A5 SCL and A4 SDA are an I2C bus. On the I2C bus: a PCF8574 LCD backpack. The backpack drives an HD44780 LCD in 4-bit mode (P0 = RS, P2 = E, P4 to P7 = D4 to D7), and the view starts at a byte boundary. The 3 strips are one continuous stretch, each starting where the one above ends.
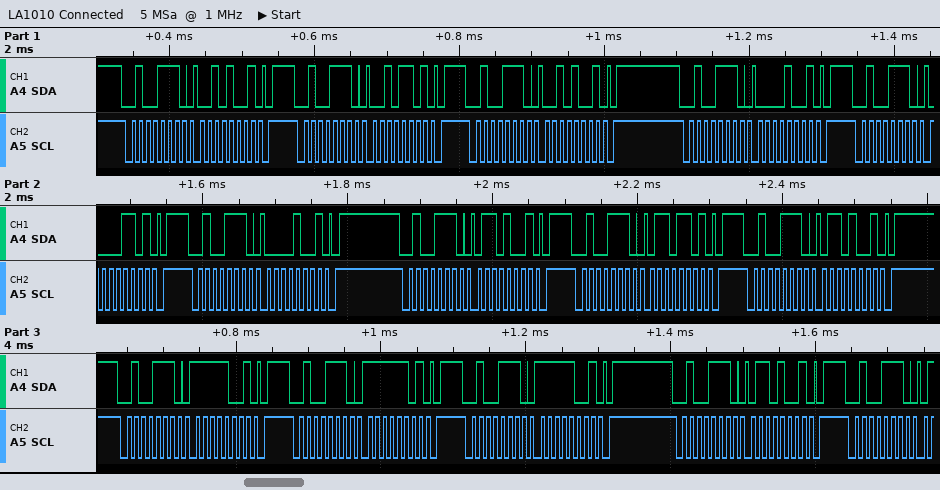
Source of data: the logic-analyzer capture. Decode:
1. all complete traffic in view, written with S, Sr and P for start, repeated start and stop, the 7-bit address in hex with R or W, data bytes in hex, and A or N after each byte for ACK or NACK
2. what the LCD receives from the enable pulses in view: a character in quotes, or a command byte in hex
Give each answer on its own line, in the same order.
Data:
S 27W A 29 A P S 27W A 2D A P S 27W A 29 A P S 27W A 09 A P S 27W A 0D A P S 27W A 09 A P S 27W A 69 A P S 27W A 6D A P S 27W A 69 A P S 27W A F9 A P S 27W A FD A P S 27W A F9 A P S 27W A 69 A P S 27W A
' ' 'o'
